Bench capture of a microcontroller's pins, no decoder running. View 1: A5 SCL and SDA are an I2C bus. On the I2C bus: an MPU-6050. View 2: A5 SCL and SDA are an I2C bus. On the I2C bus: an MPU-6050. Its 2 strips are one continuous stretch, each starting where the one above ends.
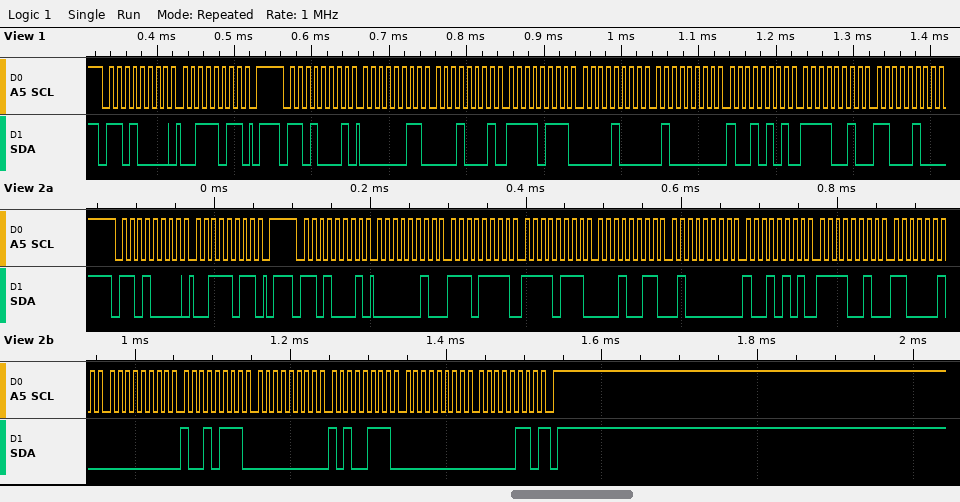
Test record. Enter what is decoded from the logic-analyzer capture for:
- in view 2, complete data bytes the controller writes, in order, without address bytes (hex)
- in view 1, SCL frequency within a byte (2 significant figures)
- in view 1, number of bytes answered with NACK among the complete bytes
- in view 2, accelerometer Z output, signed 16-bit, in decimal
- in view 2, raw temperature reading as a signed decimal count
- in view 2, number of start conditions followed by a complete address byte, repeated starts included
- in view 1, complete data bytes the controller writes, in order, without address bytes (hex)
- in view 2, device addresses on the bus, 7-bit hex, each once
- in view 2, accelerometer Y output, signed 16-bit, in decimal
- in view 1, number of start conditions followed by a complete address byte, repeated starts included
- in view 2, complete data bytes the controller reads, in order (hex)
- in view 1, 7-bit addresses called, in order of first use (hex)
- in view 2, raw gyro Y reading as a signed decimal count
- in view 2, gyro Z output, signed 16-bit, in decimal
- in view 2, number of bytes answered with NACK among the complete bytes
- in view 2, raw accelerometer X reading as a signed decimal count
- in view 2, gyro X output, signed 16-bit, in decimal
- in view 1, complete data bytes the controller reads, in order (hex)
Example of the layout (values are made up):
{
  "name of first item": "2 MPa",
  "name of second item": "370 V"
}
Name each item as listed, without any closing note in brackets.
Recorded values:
{
  "in view 2, complete data bytes the controller writes, in order, without address bytes": "3B",
  "in view 1, SCL frequency within a byte": "100 kHz",
  "in view 1, number of bytes answered with NACK among the complete bytes": "0",
  "in view 2, accelerometer Z output, signed 16-bit, in decimal": "16533",
  "in view 2, raw temperature reading as a signed decimal count": "-3390",
  "in view 2, number of start conditions followed by a complete address byte, repeated starts included": "2",
  "in view 1, complete data bytes the controller writes, in order, without address bytes": "3B",
  "in view 2, device addresses on the bus, 7-bit hex, each once": "0x68",
  "in view 2, accelerometer Y output, signed 16-bit, in decimal": "-2285",
  "in view 1, number of start conditions followed by a complete address byte, repeated starts included": "2",
  "in view 2, complete data bytes the controller reads, in order": "02 EF F7 13 40 95 F2 C2 00 97 00 A7 00 06",
  "in view 1, 7-bit addresses called, in order of first use": "0x68",
  "in view 2, raw gyro Y reading as a signed decimal count": "167",
  "in view 2, gyro Z output, signed 16-bit, in decimal": "6",
  "in view 2, number of bytes answered with NACK among the complete bytes": "1",
  "in view 2, raw accelerometer X reading as a signed decimal count": "751",
  "in view 2, gyro X output, signed 16-bit, in decimal": "151",
  "in view 1, complete data bytes the controller reads, in order": "03 11 F7 08 40 95 F2 C4"
}
